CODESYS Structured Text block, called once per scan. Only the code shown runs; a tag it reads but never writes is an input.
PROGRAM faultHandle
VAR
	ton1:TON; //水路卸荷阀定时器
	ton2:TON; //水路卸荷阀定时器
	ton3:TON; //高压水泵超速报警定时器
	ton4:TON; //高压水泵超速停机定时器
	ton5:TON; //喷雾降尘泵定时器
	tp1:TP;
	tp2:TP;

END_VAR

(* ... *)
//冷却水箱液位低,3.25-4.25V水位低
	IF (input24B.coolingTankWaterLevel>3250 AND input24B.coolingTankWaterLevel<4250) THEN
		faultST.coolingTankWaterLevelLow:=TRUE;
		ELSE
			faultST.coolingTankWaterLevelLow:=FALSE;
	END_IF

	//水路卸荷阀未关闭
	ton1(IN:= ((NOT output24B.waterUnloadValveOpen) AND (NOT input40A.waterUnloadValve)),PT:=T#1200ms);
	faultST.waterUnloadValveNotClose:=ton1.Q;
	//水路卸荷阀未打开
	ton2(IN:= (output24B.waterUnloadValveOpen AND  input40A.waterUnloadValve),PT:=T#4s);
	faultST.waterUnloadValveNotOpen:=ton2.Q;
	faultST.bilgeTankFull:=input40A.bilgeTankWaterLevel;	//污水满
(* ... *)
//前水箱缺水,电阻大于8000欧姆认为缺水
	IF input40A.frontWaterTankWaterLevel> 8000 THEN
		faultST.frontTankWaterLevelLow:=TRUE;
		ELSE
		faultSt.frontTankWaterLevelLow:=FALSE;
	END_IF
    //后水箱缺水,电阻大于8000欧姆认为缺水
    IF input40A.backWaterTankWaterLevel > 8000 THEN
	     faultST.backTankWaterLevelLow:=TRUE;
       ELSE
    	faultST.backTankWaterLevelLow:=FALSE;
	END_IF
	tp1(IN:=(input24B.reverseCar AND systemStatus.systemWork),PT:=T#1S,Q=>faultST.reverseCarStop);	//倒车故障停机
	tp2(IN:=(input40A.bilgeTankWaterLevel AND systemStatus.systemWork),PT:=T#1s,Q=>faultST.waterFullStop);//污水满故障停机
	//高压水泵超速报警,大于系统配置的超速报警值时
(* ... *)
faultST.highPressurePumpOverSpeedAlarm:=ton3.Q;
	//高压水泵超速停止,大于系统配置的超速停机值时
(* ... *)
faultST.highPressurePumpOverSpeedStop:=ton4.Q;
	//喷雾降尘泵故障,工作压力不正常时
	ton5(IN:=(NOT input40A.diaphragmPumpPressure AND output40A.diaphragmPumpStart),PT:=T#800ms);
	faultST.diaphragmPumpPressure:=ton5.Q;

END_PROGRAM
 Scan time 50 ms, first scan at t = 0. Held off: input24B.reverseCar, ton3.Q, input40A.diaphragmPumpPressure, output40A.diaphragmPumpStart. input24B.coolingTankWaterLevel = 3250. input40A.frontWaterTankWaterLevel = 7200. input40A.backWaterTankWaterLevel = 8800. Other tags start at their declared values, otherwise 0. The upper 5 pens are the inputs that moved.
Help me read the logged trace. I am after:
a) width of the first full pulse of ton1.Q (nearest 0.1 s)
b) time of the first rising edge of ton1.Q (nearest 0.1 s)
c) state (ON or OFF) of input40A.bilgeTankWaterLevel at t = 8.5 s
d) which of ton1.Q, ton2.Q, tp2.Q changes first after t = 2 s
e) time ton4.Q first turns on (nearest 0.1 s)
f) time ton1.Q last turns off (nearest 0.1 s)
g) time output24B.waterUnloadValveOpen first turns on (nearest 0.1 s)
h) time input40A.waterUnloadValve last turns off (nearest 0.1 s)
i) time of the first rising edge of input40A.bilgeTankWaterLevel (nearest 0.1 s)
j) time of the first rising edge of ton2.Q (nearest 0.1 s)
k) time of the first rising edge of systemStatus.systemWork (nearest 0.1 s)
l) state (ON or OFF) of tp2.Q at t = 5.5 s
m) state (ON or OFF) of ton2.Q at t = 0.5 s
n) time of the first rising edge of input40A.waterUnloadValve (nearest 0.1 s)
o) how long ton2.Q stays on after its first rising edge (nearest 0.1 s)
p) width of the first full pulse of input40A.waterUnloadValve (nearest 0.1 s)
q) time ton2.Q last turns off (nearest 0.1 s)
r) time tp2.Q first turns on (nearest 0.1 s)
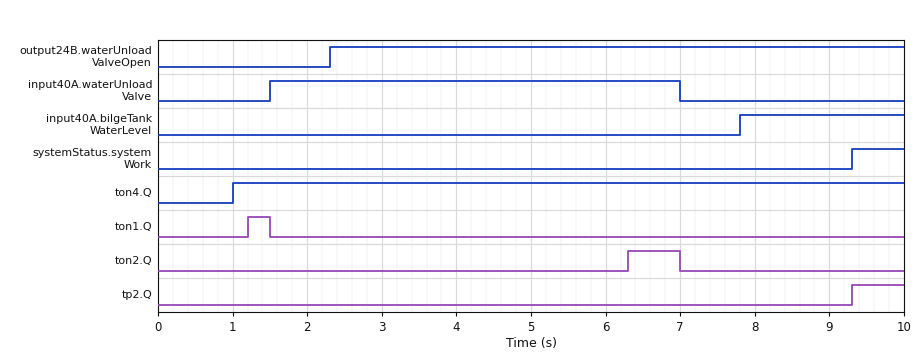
0.3 s
1.2 s
ON
ton2.Q
1.0 s
1.5 s
2.3 s
7.0 s
7.8 s
6.3 s
9.3 s
OFF
OFF
1.5 s
0.7 s
5.5 s
7.0 s
9.3 s
